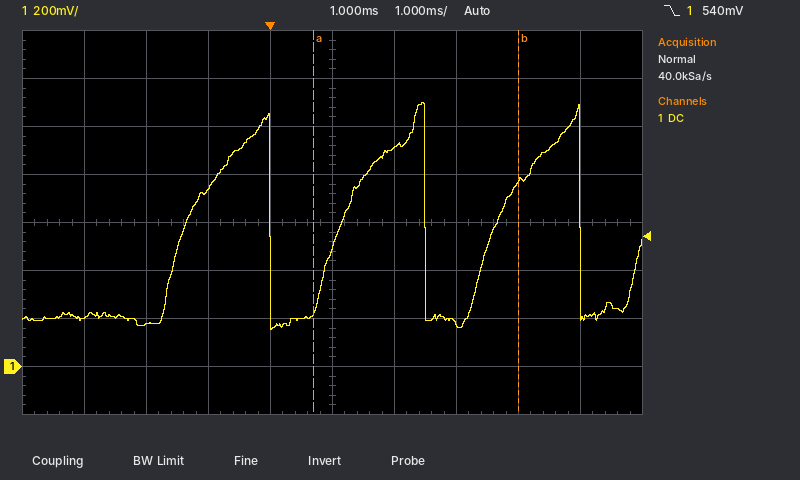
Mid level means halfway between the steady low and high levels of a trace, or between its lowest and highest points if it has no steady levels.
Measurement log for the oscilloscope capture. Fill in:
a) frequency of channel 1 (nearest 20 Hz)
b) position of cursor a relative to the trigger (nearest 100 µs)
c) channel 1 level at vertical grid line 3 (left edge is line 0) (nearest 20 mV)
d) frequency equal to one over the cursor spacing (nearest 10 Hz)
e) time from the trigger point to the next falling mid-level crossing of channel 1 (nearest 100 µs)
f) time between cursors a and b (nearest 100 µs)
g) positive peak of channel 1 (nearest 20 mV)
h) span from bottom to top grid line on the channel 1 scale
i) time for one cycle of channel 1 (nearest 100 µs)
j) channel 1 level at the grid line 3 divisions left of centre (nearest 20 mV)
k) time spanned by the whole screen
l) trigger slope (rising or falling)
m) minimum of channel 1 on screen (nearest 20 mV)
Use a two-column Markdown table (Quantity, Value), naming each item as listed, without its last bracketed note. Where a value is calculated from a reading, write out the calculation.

| Quantity | Value |
|---|---|
| frequency of channel 1 | 1 / 2.5 ms ≈ 400 Hz |
| position of cursor a relative to the trigger | +700 µs |
| channel 1 level at vertical grid line 3 (left edge is line 0) | 740 mV |
| frequency equal to one over the cursor spacing | 1 / 3.3 ms ≈ 300 Hz |
| time from the trigger point to the next falling mid-level crossing of channel 1 | 2.5 ms |
| time between cursors a and b | 3.3 ms |
| positive peak of channel 1 | 1.10 V |
| span from bottom to top grid line on the channel 1 scale | 1.6 V |
| time for one cycle of channel 1 | 2.5 ms |
| channel 1 level at the grid line 3 divisions left of centre | 180 mV |
| time spanned by the whole screen | 10 ms |
| trigger slope | falling |
| minimum of channel 1 on screen | 160 mV |
